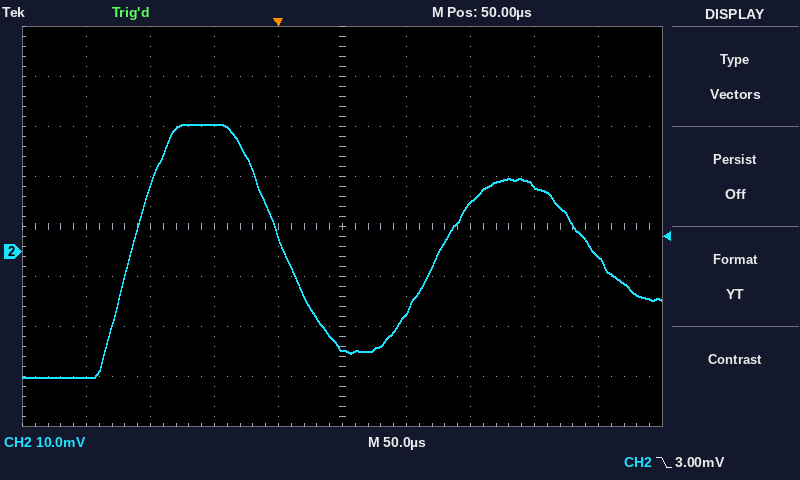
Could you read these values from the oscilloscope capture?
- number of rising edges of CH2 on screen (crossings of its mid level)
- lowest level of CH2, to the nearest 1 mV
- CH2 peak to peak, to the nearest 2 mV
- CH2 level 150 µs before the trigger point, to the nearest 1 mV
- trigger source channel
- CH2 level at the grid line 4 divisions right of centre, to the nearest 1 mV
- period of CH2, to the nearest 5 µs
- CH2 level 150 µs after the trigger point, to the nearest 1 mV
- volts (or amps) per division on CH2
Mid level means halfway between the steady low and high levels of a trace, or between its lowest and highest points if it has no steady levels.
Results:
2
-25 mV
50 mV
-25 mV
CH2
-1 mV
240 µs
10 mV
10 mV
